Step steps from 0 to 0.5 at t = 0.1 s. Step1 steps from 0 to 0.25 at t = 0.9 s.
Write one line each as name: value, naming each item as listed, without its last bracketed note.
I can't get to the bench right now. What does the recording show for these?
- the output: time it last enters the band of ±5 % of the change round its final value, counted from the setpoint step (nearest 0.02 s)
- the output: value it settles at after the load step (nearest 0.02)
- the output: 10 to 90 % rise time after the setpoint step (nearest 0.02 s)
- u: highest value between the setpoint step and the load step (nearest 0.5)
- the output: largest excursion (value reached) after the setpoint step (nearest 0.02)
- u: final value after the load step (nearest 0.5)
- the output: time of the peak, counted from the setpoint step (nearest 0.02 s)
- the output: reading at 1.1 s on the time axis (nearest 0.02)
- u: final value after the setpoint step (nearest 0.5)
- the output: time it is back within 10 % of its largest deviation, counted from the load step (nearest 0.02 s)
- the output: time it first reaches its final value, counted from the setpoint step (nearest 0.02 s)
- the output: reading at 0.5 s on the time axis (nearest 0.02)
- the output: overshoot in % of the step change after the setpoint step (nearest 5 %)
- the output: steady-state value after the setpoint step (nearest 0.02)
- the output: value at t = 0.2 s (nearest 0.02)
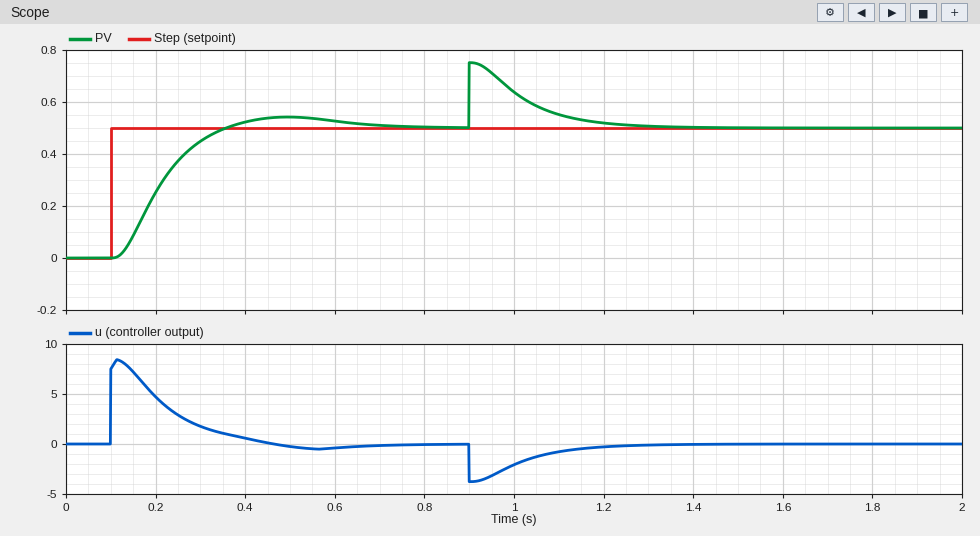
the output: time it last enters the band of ±5 % of the change round its final value, counted from the setpoint step: 0.50 s
the output: value it settles at after the load step: 0.50
the output: 10 to 90 % rise time after the setpoint step: 0.16 s
u: highest value between the setpoint step and the load step: 8.5
the output: largest excursion (value reached) after the setpoint step: 0.54
u: final value after the load step: 0.0
the output: time of the peak, counted from the setpoint step: 0.40 s
the output: reading at 1.1 s on the time axis: 0.56
u: final value after the setpoint step: 0.0
the output: time it is back within 10 % of its largest deviation, counted from the load step: 0.28 s
the output: time it first reaches its final value, counted from the setpoint step: 0.26 s
the output: reading at 0.5 s on the time axis: 0.54
the output: overshoot in % of the step change after the setpoint step: 10 %
the output: steady-state value after the setpoint step: 0.50
the output: value at t = 0.2 s: 0.26
